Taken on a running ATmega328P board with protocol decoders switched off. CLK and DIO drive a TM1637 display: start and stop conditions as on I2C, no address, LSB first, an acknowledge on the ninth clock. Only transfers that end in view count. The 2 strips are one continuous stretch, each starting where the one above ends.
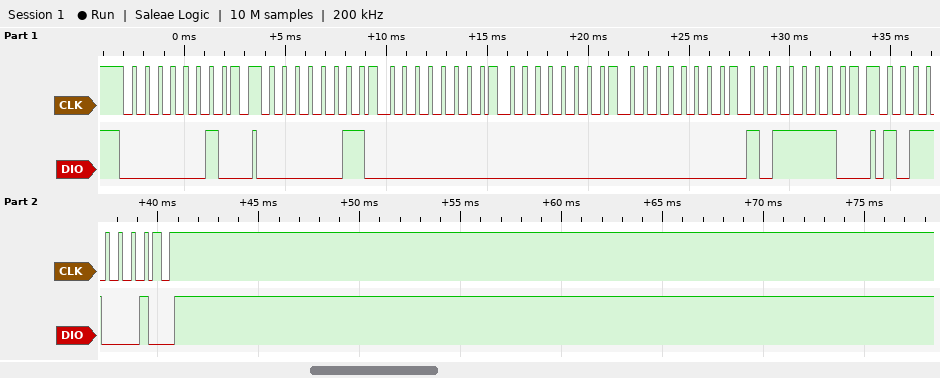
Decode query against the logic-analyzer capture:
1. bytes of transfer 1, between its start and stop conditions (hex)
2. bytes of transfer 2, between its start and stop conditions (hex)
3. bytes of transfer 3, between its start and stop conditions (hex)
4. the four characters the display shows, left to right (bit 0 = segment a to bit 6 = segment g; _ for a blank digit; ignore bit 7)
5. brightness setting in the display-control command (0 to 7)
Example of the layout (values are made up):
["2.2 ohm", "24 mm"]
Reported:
["40", "C0 00 00 00 7D", "8D", "___6", "5"]
